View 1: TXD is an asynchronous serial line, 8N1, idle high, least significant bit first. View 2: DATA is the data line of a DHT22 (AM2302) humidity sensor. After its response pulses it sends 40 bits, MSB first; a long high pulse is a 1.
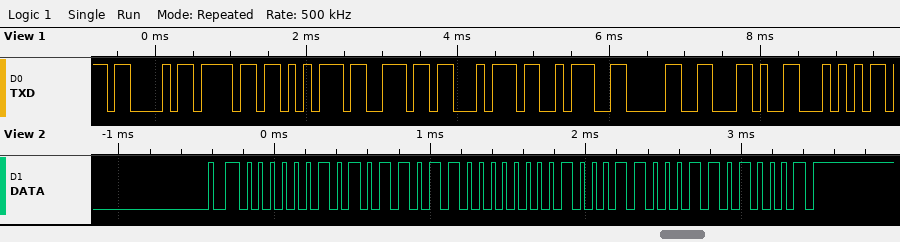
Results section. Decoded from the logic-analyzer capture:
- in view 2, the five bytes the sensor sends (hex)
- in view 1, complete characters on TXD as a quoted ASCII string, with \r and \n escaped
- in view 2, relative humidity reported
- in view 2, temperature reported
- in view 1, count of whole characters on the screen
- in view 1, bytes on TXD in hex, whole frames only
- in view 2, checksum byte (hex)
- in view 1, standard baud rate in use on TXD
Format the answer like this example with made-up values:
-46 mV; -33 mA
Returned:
02 B6 01 18 D1; "Count:0,T"; 69.4 %; 28.0 °C; 9; 43 6F 75 6E 74 3A 30 2C 54; 0xD1; 9600 baud
